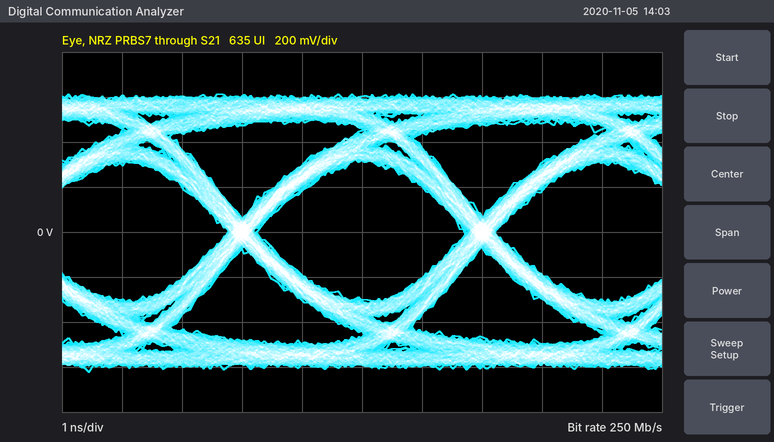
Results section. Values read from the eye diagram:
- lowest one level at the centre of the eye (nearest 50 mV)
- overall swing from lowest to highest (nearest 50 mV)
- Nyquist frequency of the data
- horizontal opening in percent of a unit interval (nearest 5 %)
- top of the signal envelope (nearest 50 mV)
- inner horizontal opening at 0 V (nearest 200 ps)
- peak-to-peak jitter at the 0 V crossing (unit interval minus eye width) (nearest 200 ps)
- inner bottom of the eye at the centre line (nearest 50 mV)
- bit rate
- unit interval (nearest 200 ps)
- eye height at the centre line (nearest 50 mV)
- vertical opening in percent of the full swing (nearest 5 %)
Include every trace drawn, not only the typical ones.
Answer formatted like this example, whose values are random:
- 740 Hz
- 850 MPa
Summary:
- 300 mV
- 1.25 V
- 125 MHz
- 85 %
- 600 mV
- 3.4 ns
- 600 ps
- -300 mV
- 250 Mb/s
- 4.0 ns
- 600 mV
- 50 %
